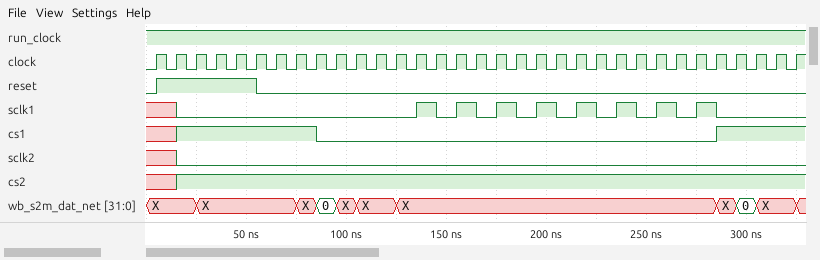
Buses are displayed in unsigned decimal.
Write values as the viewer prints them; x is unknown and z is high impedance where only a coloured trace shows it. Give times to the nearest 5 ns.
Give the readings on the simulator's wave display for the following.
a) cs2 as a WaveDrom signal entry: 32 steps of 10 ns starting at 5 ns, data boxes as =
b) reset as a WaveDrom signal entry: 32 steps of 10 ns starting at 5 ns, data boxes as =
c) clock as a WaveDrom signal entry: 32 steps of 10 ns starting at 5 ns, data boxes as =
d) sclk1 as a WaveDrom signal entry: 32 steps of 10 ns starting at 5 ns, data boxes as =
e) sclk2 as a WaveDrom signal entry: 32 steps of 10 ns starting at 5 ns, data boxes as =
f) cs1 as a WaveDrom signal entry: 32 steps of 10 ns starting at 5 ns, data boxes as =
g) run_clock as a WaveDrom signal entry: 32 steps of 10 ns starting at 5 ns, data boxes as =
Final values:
{name: 'cs2', wave: 'x1..............................'}
{name: 'reset', wave: '1....0..........................'}
{name: 'clock', wave: 'p...............................'}
{name: 'sclk1', wave: 'x0...........1010101010101010...'}
{name: 'sclk2', wave: 'x0..............................'}
{name: 'cs1', wave: 'x1......0...................1...'}
{name: 'run_clock', wave: '1...............................'}
